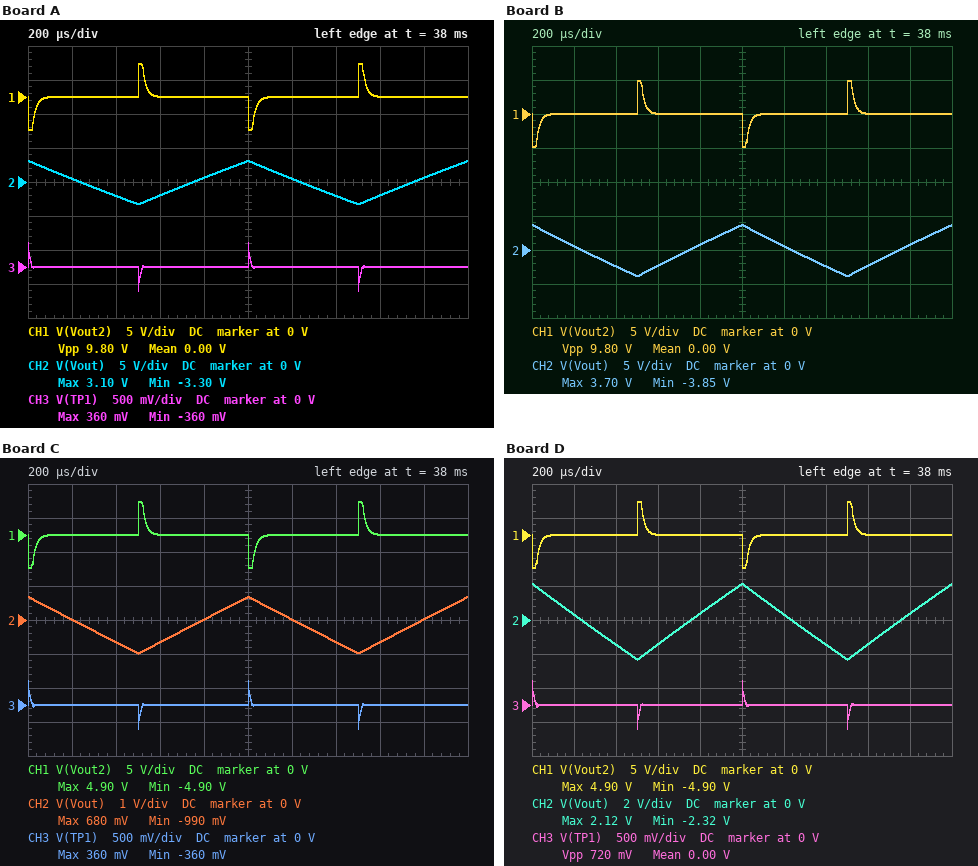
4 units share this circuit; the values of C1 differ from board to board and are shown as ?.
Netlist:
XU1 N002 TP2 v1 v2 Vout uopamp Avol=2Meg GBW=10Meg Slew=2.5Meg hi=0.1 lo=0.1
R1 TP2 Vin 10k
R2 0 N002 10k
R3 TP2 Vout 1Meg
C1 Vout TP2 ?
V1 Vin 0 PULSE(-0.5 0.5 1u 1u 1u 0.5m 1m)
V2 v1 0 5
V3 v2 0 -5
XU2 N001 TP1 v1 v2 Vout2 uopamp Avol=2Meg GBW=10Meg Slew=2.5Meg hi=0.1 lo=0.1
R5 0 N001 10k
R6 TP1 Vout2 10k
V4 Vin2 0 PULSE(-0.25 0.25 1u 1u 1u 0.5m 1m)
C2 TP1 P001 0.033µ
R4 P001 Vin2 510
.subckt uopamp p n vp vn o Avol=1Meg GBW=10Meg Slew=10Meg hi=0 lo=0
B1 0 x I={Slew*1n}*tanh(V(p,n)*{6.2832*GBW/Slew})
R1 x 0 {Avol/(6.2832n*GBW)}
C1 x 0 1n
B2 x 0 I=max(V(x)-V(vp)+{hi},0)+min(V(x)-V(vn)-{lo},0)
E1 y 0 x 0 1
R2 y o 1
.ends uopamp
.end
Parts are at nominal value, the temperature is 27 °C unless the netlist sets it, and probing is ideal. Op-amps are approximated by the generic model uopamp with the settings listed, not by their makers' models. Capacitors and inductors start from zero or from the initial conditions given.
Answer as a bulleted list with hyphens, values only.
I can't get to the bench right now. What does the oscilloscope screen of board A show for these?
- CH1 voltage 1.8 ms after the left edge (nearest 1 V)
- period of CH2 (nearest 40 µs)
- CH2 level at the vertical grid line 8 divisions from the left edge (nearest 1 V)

- 0 V
- 1.00 ms
- -2 V
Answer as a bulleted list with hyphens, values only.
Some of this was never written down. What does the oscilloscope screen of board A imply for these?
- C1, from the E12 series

- 3.9 nF
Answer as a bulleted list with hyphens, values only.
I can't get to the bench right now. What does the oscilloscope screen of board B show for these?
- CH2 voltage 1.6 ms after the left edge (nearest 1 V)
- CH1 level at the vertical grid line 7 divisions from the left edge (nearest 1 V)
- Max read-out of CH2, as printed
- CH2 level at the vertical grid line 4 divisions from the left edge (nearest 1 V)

- -2 V
- 0 V
- 3.70 V
- 1 V
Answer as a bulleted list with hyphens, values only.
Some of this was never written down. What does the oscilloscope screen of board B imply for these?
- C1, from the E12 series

- 3.3 nF
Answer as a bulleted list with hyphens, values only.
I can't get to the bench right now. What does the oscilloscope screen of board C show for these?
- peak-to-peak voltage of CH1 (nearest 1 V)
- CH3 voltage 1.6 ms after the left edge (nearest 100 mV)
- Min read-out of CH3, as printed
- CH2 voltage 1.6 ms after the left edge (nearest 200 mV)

- 10 V
- 0 V
- -360 mV
- -600 mV
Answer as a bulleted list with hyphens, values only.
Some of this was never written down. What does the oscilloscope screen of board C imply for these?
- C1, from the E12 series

- 15 nF
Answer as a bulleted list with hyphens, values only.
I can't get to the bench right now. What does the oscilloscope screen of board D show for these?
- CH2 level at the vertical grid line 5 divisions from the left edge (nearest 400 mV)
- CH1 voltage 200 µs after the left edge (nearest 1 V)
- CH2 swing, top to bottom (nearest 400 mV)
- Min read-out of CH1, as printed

- 2.0 V
- 0 V
- 4.4 V
- -4.90 V
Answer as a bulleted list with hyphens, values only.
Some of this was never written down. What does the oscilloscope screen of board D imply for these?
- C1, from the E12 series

- 5.6 nF
